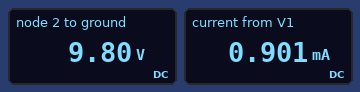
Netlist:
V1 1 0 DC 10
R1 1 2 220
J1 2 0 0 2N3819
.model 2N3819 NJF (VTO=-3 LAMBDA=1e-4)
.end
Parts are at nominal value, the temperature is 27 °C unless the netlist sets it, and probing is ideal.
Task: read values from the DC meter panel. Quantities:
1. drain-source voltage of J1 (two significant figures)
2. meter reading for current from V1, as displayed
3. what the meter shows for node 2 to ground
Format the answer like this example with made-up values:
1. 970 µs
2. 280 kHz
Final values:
1. 9.8 V
2. 0.901 mA
3. 9.80 V
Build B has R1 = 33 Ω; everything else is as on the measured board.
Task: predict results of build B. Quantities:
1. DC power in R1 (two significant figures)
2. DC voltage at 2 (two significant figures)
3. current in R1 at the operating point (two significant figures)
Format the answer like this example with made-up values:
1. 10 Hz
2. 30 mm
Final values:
1. 27 µW
2. 10 V
3. 900 µA
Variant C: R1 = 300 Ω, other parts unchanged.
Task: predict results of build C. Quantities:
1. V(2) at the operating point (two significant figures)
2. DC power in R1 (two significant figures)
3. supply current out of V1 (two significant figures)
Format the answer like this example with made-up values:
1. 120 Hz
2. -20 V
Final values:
1. 9.7 V
2. 240 µW
3. 900 µA
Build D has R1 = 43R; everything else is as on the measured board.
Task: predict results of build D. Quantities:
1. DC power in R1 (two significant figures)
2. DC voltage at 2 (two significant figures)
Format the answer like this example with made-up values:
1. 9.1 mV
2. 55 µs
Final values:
1. 35 µW
2. 10 V
